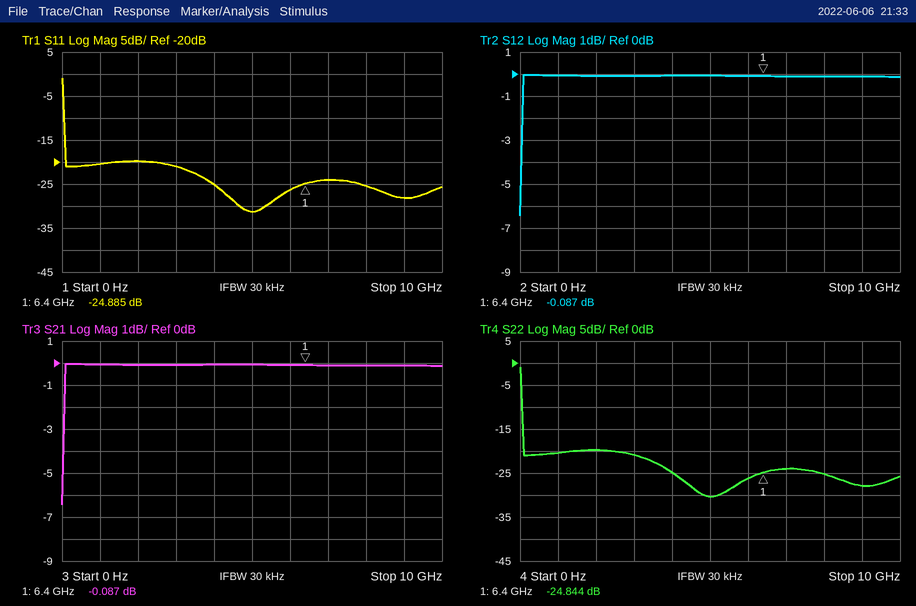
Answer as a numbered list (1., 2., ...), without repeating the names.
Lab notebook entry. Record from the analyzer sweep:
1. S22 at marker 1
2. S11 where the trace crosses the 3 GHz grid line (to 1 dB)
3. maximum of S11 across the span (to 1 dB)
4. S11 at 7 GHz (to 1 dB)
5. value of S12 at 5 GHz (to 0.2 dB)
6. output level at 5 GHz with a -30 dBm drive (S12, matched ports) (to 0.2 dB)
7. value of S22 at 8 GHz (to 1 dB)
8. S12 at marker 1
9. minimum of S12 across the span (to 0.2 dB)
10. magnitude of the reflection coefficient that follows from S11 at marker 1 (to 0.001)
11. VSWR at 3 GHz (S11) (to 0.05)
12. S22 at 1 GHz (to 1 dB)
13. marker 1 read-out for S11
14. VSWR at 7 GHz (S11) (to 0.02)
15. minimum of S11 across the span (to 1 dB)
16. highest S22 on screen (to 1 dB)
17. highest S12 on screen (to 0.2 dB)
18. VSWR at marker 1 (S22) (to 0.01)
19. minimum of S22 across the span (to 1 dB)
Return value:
1. -24.844 dB
2. -21 dB
3. -1 dB
4. -24 dB
5. 0.0 dB
6. -30.0 dBm
7. -25 dB
8. -0.087 dB
9. -6.4 dB
10. 0.057
11. 1.20
12. -20 dB
13. -24.885 dB
14. 1.14
15. -31 dB
16. -1 dB
17. 0.0 dB
18. 1.12
19. -30 dB
